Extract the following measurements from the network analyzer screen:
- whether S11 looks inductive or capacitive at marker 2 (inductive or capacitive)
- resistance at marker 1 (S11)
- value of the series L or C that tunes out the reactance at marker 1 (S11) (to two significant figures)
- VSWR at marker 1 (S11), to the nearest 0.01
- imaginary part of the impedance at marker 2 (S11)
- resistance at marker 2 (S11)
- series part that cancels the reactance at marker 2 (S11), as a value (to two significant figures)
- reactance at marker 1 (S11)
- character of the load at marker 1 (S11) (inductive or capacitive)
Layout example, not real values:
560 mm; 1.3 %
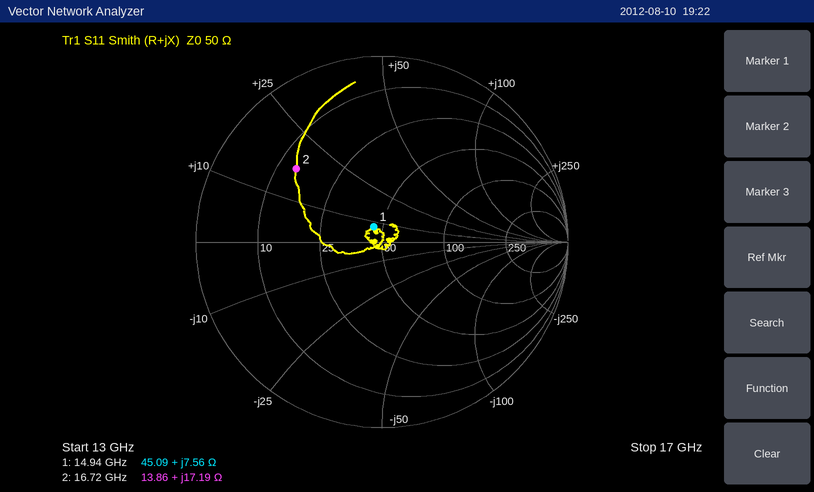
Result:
inductive; 45.09 Ω; 1.4 pF; 1.21; +17.19 Ω; 13.86 Ω; 550 fF; +7.56 Ω; inductive
